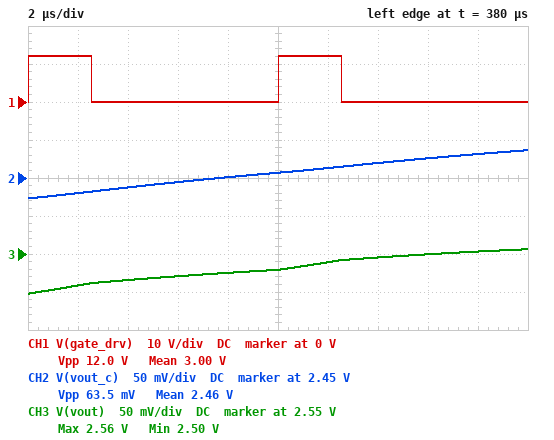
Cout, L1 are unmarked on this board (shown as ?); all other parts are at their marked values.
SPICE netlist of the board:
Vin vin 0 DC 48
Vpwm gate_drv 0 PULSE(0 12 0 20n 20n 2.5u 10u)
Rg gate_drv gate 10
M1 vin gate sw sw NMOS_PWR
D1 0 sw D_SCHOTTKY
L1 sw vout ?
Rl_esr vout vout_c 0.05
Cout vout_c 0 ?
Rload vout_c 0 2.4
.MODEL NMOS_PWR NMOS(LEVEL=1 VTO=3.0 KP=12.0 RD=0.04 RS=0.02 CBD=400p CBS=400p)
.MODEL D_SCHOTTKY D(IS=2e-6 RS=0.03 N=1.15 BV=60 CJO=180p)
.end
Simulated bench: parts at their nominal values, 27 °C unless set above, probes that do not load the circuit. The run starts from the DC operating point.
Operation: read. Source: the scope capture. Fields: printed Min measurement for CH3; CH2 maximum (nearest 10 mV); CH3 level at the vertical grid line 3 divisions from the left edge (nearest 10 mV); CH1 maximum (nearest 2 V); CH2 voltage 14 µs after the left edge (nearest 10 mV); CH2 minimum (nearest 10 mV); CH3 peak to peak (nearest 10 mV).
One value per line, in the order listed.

2.50 V
2.49 V
2.52 V
12 V
2.47 V
2.42 V
60 mV
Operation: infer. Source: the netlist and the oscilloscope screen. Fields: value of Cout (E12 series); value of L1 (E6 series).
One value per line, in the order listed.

150 µF
150 µH
